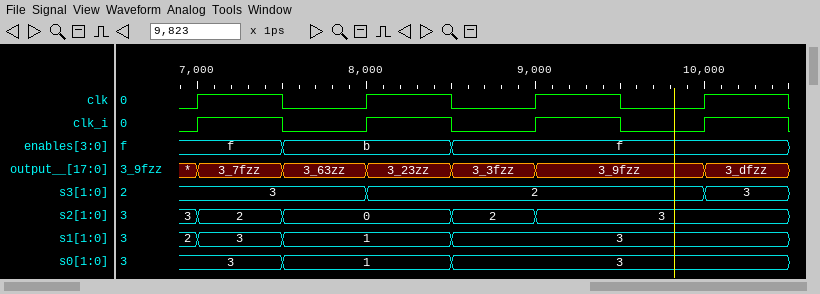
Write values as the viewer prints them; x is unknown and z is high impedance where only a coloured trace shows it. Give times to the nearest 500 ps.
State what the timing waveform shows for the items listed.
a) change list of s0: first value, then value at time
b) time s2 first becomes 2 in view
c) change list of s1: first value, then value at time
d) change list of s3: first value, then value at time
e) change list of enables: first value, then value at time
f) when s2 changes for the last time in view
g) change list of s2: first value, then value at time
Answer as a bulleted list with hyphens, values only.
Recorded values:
- 3, 1 at 7500 ps, 3 at 8500 ps
- 7000 ps
- 2, 3 at 7000 ps, 1 at 7500 ps, 3 at 8500 ps
- 3, 2 at 8000 ps, 3 at 10000 ps
- f, b at 7500 ps, f at 8500 ps
- 9000 ps
- 3, 2 at 7000 ps, 0 at 7500 ps, 2 at 8500 ps, 3 at 9000 ps
